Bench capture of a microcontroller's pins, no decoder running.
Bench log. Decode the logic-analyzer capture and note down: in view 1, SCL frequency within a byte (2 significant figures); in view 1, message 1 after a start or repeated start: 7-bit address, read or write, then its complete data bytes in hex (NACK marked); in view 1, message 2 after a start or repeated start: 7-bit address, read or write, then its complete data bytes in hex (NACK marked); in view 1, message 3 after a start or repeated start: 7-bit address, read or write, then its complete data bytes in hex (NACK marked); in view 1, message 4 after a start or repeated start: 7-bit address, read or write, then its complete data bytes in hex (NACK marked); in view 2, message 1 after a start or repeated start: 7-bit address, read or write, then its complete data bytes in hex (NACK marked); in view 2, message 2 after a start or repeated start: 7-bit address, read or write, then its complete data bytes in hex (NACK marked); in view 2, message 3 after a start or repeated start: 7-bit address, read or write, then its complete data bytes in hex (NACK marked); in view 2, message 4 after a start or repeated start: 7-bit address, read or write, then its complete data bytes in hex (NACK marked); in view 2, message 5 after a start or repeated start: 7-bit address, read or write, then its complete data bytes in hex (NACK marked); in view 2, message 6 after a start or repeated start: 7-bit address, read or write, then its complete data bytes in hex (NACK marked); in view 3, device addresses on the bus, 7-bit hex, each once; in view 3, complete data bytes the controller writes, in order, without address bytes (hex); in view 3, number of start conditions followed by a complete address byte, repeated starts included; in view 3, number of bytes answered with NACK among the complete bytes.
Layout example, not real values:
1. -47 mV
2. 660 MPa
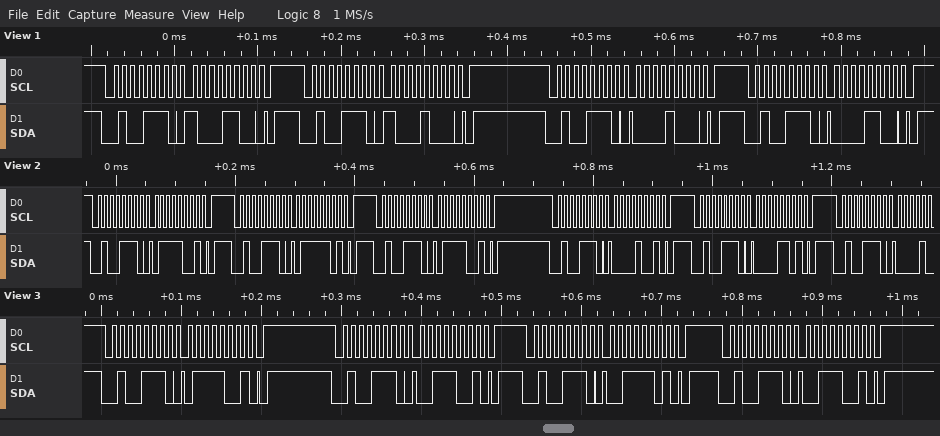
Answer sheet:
1. 100 kHz
2. 0x27 write: 8C
3. 0x27 write: 88
4. 0x27 write: 08
5. 0x27 write: 0C
6. 0x27 write: 79
7. 0x27 write: 7D
8. 0x27 write: 79
9. 0x27 write: 09
10. 0x27 write: 0D
11. 0x27 write
12. 0x27
13. 79 39 3D 39
14. 4
15. 0
